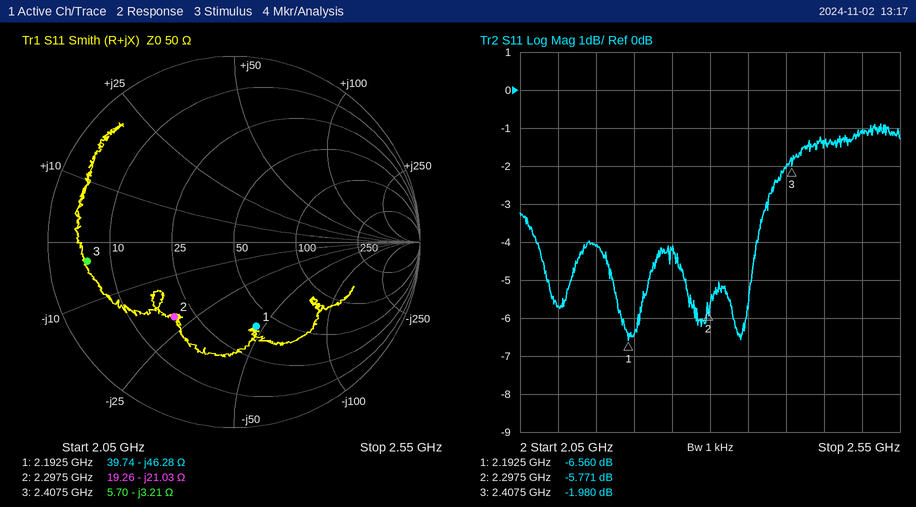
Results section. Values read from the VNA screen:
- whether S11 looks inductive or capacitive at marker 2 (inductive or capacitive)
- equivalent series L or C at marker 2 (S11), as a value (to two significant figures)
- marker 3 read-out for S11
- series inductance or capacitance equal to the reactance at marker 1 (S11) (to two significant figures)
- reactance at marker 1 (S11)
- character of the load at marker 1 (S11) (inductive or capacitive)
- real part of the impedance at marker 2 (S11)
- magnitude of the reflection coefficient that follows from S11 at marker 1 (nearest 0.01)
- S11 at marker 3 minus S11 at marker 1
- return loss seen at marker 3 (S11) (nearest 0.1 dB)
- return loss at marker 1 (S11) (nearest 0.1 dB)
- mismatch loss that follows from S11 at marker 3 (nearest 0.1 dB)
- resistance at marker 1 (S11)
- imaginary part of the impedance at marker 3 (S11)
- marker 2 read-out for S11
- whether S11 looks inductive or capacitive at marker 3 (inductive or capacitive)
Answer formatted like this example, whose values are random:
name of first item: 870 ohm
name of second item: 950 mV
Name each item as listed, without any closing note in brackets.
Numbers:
whether S11 looks inductive or capacitive at marker 2: capacitive
equivalent series L or C at marker 2 (S11), as a value: 3.3 pF
marker 3 read-out for S11: -1.980 dB
series inductance or capacitance equal to the reactance at marker 1 (S11): 1.6 pF
reactance at marker 1: -46.28 Ω
character of the load at marker 1 (S11): capacitive
real part of the impedance at marker 2: 19.26 Ω
magnitude of the reflection coefficient that follows from S11 at marker 1: 0.47
S11 at marker 3 minus S11 at marker 1: 4.580 dB
return loss seen at marker 3 (S11): 2.0 dB
return loss at marker 1 (S11): 6.6 dB
mismatch loss that follows from S11 at marker 3: 4.4 dB
resistance at marker 1: 39.74 Ω
imaginary part of the impedance at marker 3: -3.21 Ω
marker 2 read-out for S11: -5.771 dB
whether S11 looks inductive or capacitive at marker 3: capacitive
